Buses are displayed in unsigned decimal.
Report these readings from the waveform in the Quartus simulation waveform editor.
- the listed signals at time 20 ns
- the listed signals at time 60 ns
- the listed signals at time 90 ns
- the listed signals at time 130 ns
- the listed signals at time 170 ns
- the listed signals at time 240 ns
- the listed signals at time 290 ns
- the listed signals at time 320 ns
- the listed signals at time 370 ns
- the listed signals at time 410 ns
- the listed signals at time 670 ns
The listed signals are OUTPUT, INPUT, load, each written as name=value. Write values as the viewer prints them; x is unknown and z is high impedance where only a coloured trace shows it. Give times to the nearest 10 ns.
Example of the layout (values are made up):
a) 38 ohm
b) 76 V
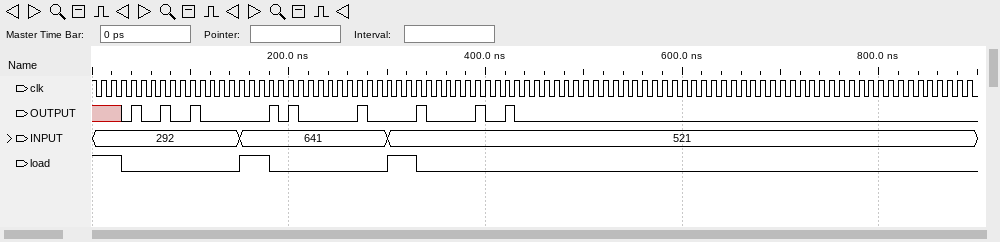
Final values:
a) OUTPUT=x, INPUT=292, load=1
b) OUTPUT=0, INPUT=292, load=0
c) OUTPUT=0, INPUT=292, load=0
d) OUTPUT=0, INPUT=292, load=0
e) OUTPUT=0, INPUT=641, load=1
f) OUTPUT=0, INPUT=641, load=0
g) OUTPUT=0, INPUT=641, load=0
h) OUTPUT=0, INPUT=521, load=1
i) OUTPUT=0, INPUT=521, load=0
j) OUTPUT=0, INPUT=521, load=0
k) OUTPUT=0, INPUT=521, load=0
